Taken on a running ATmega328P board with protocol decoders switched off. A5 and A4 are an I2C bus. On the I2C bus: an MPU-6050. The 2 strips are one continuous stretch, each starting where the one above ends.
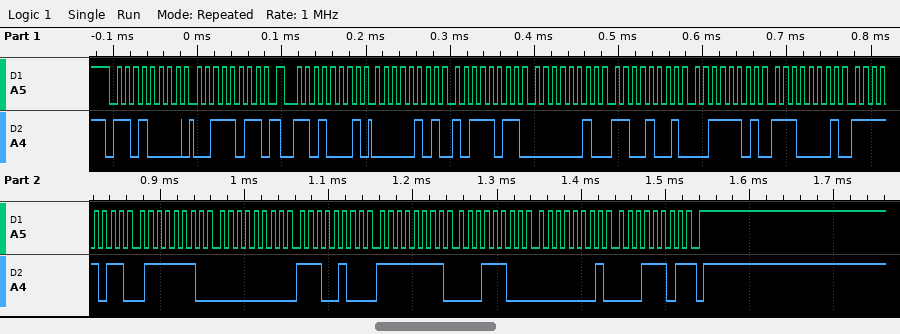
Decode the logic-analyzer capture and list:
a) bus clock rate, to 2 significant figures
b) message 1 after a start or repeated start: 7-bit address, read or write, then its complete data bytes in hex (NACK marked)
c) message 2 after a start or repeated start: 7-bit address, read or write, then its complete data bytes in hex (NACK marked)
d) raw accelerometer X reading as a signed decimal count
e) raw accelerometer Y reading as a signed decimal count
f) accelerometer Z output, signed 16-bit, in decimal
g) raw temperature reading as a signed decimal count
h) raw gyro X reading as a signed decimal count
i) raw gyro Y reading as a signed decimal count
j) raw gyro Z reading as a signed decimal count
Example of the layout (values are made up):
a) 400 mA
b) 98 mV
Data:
a) 100 kHz
b) 0x68 write: 3B
c) 0x68 read: 05 BB 02 C9 3D E1 FB 7E 00 E4 FF 1C 01 1D NACK
d) 1467
e) 713
f) 15841
g) -1154
h) 228
i) -228
j) 285
